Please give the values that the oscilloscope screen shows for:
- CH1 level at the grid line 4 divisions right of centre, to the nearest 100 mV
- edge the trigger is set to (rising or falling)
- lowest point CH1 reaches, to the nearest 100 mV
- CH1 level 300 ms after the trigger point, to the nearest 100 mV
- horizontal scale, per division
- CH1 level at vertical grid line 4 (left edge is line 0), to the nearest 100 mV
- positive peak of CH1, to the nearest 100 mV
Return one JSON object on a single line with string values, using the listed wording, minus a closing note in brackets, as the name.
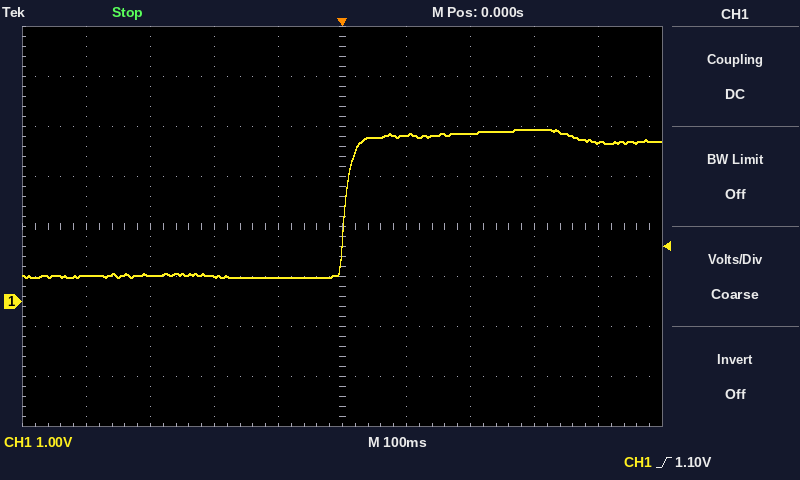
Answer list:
{"CH1 level at the grid line 4 divisions right of centre, to the nearest 100 mV": "3.2 V", "edge the trigger is set to": "rising", "lowest point CH1 reaches, to the nearest 100 mV": "500 mV", "CH1 level 300 ms after the trigger point, to the nearest 100 mV": "3.4 V", "horizontal scale, per division": "100 ms", "CH1 level at vertical grid line 4 (left edge is line 0), to the nearest 100 mV": "500 mV", "positive peak of CH1, to the nearest 100 mV": "3.4 V"}
